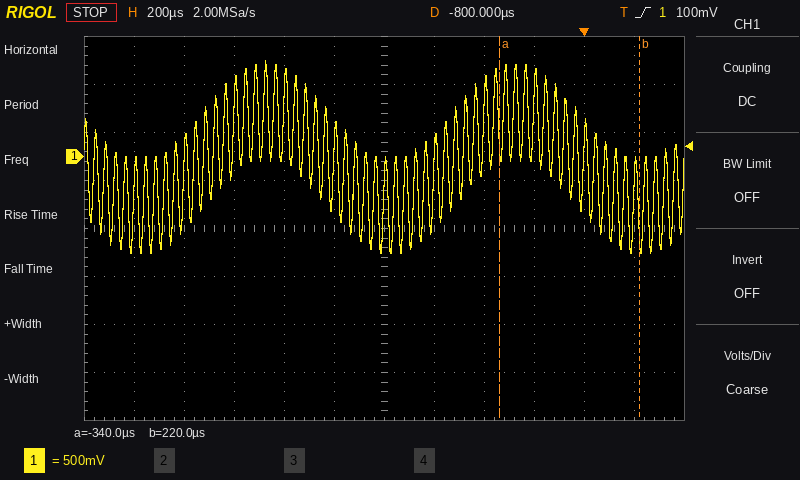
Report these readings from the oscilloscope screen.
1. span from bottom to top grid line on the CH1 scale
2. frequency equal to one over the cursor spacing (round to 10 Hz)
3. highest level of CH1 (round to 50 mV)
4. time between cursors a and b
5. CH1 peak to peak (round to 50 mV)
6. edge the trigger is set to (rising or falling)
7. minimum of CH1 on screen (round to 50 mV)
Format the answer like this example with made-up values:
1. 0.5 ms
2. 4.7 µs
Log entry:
1. 4 V
2. 1.79 kHz
3. 1.00 V
4. 560 µs
5. 2.00 V
6. rising
7. -1.00 V
